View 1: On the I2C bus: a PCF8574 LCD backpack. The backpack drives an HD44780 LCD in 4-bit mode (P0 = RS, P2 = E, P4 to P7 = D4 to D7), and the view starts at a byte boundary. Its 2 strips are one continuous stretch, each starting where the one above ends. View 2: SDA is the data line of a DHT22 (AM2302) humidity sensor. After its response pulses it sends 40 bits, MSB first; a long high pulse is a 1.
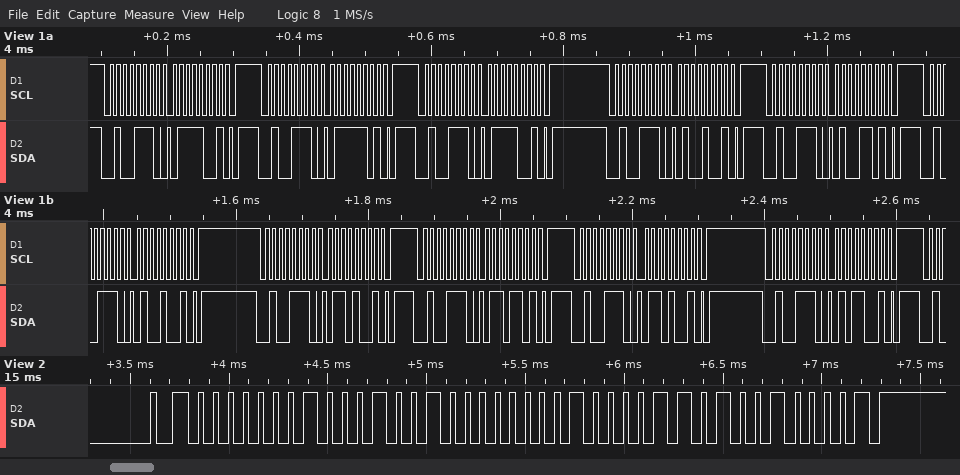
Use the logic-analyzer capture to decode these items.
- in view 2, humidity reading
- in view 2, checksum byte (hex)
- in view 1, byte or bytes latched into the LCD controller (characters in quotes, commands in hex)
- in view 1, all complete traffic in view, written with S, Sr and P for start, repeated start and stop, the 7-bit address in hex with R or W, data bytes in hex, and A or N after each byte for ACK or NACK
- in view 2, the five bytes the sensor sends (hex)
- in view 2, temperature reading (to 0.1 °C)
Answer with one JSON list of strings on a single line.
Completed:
["27.4 %", "0x21", "'t'", "S 27W A 79 A P S 27W A 7D A P S 27W A 79 A P S 27W A 49 A P S 27W A 4D A P S 27W A 49 A P S 27W A 69 A P S 27W A 6D A P S 27W A 69 A P S 27W A 59 A P", "01 12 01 0D 21", "26.9 °C"]
